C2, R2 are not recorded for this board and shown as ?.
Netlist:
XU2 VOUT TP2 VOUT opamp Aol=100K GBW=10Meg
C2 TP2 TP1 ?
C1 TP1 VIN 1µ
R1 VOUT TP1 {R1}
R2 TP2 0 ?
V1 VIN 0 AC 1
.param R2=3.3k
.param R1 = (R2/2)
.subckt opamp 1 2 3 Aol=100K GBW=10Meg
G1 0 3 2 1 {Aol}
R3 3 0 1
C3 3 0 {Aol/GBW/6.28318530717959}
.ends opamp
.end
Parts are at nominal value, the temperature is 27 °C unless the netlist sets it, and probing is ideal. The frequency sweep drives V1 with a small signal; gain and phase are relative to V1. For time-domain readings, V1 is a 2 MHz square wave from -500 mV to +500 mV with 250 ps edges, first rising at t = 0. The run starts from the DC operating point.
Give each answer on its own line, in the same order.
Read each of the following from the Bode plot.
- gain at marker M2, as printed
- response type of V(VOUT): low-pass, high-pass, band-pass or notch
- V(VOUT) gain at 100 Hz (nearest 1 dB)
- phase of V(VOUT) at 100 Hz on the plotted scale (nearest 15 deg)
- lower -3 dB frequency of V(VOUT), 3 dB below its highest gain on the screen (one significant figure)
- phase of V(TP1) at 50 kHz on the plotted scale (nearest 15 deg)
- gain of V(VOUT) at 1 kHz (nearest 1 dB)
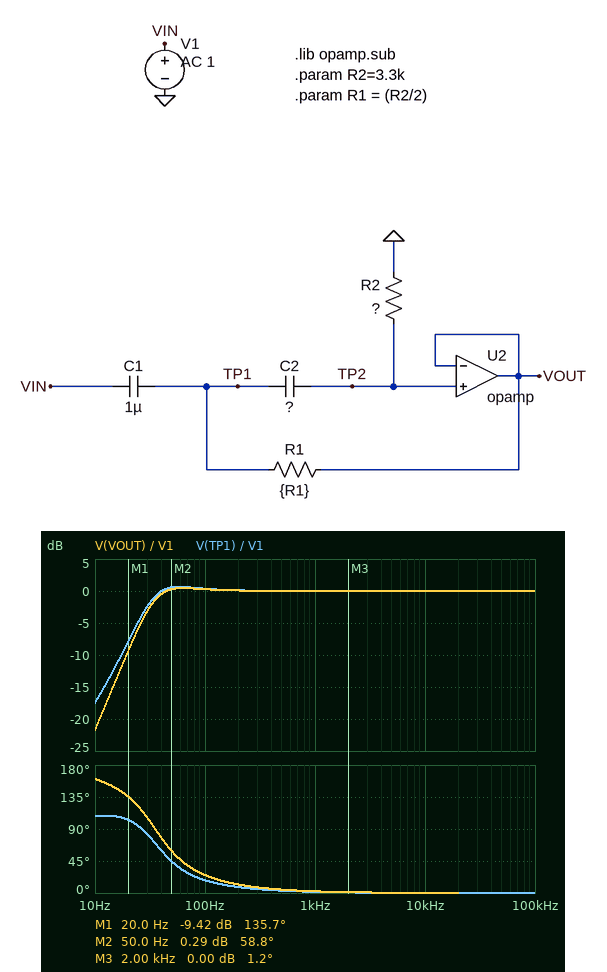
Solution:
0.29 dB
high-pass
0 dB
30 deg
30 Hz
0 deg
0 dB
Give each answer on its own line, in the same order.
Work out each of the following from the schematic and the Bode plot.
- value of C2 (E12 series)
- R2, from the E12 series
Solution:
2.2 µF
5.6 kΩ
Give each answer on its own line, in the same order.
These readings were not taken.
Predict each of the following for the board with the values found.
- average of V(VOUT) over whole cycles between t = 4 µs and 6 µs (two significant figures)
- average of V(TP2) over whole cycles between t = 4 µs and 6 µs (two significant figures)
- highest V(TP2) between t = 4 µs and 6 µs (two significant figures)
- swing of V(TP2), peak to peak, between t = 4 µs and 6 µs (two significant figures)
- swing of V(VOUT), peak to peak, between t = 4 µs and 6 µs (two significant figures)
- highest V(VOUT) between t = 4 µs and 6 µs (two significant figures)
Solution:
500 mV
500 mV
1.0 V
1.0 V
1.0 V
1.0 V
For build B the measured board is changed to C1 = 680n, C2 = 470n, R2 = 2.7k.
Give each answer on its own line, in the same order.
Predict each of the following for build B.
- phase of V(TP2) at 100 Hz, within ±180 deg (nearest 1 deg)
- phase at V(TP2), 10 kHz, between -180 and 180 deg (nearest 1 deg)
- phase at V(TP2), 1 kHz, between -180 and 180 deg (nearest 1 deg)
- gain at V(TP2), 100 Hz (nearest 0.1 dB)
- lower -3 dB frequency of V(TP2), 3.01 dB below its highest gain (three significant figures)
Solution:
110 deg
1 deg
12 deg
-7.1 dB
152 Hz
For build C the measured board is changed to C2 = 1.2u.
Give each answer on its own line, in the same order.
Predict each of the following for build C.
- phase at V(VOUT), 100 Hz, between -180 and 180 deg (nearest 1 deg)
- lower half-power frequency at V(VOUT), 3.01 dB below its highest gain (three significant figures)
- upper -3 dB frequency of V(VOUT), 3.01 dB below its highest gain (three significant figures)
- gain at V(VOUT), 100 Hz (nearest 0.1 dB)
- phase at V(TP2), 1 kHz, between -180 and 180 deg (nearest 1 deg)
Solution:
34 deg
41.6 Hz
8.19 MHz
0.6 dB
3 deg
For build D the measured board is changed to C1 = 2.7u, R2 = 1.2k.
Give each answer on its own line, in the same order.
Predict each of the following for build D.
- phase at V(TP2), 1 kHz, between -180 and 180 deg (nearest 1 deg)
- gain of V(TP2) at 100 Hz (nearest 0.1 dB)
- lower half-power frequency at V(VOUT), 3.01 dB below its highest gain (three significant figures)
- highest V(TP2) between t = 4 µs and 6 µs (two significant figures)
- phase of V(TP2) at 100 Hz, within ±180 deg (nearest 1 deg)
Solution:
6 deg
-2.6 dB
90.7 Hz
1.0 V
54 deg
